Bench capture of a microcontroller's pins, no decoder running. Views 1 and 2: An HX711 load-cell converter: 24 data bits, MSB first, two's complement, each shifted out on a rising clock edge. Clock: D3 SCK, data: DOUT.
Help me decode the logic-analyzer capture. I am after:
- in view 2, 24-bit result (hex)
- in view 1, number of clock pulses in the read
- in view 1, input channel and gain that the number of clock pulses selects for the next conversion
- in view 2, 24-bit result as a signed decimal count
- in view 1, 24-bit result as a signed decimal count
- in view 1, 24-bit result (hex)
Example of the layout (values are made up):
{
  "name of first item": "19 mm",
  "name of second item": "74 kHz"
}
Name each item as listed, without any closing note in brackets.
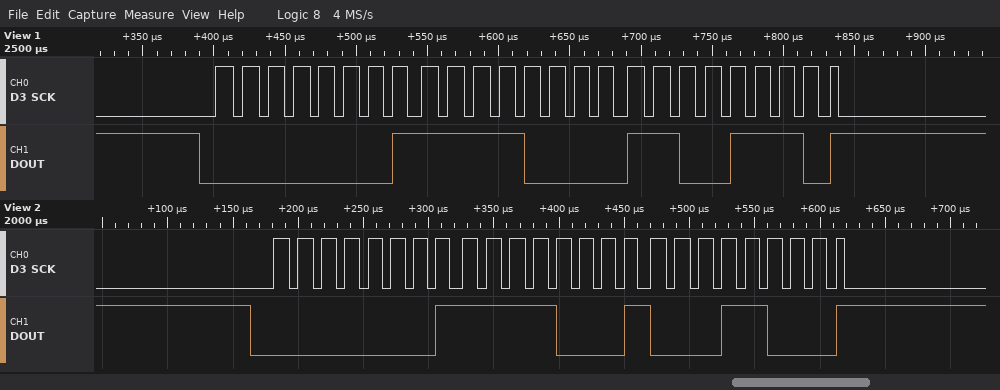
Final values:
{
  "in view 2, 24-bit result": "0x01F118",
  "in view 1, number of clock pulses in the read": "25",
  "in view 1, input channel and gain that the number of clock pulses selects for the next conversion": "channel A, gain 128",
  "in view 2, 24-bit result as a signed decimal count": "127256",
  "in view 1, 24-bit result as a signed decimal count": "127182",
  "in view 1, 24-bit result": "0x01F0CE"
}
